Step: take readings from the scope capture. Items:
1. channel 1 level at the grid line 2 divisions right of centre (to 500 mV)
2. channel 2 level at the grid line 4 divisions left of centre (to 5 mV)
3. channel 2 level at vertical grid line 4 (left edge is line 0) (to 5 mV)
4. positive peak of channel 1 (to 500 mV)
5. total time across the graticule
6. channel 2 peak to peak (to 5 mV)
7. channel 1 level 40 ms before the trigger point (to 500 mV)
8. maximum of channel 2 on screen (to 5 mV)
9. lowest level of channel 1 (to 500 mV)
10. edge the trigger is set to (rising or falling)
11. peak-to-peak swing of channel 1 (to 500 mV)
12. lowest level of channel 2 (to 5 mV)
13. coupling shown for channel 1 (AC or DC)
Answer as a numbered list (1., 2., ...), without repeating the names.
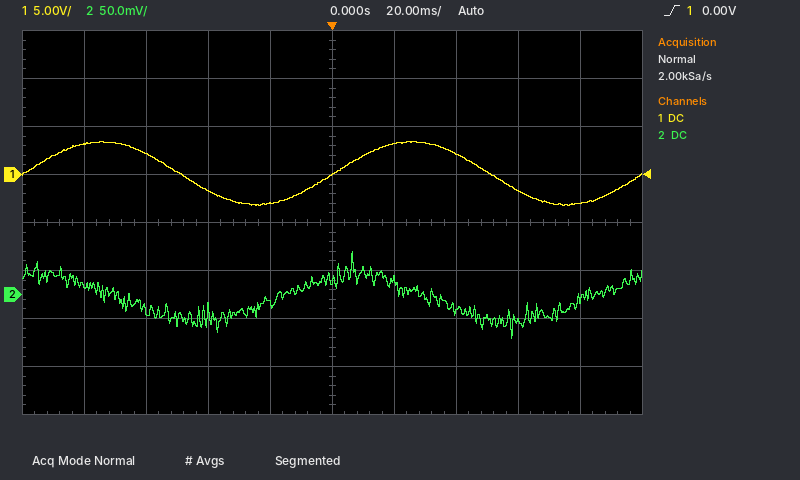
1. 2.0 V
2. 10 mV
3. -10 mV
4. 3.5 V
5. 200 ms
6. 90 mV
7. -1.5 V
8. 45 mV
9. -3.0 V
10. rising
11. 6.5 V
12. -45 mV
13. DC
